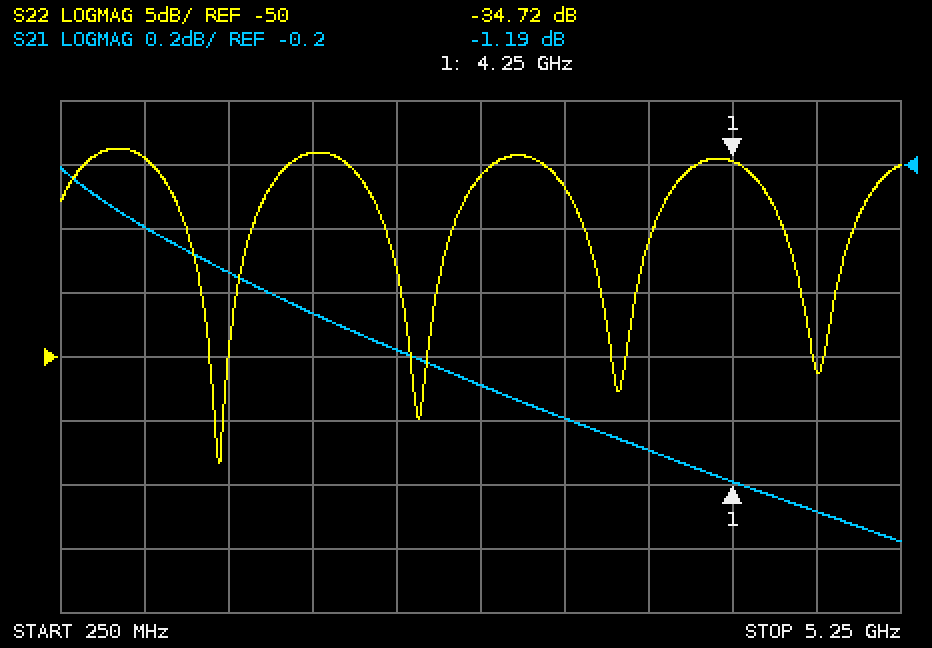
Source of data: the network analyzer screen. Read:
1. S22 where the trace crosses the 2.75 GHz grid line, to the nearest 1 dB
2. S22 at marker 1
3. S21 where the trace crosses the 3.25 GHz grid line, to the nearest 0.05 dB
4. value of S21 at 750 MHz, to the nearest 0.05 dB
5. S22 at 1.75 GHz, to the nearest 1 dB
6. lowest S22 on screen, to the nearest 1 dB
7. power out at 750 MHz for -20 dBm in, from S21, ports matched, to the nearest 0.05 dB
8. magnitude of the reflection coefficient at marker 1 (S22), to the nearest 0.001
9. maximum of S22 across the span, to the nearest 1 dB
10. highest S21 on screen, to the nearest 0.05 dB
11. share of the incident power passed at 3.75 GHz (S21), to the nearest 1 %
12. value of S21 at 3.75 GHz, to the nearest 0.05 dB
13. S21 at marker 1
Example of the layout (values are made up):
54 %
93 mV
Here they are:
-36 dB
-34.72 dB
-1.00 dB
-0.40 dB
-34 dB
-58 dB
-20.40 dBm
0.018
-34 dB
-0.20 dB
78 %
-1.10 dB
-1.19 dB
